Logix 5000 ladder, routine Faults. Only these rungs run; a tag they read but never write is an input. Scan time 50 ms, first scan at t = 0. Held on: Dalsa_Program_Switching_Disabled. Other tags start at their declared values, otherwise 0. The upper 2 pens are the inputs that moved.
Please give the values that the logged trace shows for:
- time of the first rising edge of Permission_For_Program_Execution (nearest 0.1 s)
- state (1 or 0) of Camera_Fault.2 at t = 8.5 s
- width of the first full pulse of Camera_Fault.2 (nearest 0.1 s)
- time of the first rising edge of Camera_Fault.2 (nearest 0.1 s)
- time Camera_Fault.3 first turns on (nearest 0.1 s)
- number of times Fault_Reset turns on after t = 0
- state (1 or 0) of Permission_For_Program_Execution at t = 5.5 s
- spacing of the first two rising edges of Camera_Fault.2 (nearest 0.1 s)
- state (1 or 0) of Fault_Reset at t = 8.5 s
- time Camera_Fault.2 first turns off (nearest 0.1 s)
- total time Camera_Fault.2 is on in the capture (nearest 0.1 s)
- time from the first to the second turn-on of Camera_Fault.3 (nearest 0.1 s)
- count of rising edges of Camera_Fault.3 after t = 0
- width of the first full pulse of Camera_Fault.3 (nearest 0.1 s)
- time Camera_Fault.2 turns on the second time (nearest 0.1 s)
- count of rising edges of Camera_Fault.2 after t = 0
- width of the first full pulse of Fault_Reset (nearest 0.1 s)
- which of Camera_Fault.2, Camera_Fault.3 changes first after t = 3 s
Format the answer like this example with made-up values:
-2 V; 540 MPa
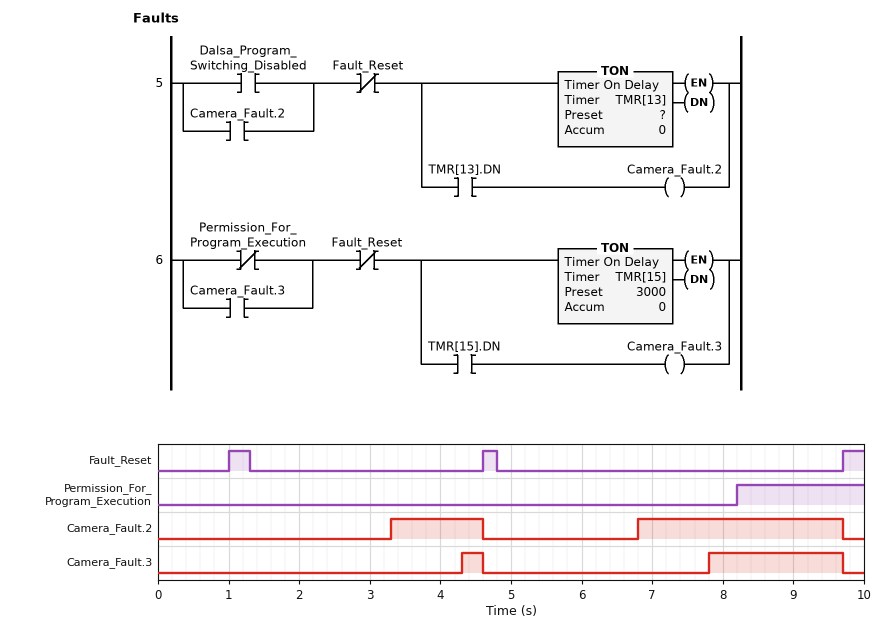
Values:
8.2 s; 1; 1.3 s; 3.3 s; 4.3 s; 3; 0; 3.5 s; 0; 4.6 s; 4.2 s; 3.5 s; 2; 0.3 s; 6.8 s; 2; 0.3 s; Camera_Fault.2
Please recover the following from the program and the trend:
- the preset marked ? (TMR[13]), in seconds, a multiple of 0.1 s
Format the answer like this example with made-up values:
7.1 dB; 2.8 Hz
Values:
2.0 s
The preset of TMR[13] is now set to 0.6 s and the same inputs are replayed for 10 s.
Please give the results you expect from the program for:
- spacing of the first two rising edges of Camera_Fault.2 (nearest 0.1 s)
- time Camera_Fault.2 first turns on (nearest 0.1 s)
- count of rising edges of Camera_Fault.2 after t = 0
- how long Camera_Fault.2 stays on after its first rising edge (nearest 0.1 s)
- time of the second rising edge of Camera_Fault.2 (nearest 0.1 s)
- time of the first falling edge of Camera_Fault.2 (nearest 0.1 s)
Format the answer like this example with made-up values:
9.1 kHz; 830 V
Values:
1.3 s; 0.6 s; 3; 0.4 s; 1.9 s; 1.0 s
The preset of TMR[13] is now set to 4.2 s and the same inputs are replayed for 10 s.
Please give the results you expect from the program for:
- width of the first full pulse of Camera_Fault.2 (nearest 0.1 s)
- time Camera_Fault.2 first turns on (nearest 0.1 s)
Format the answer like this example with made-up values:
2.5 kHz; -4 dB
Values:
0.7 s; 9.0 s
